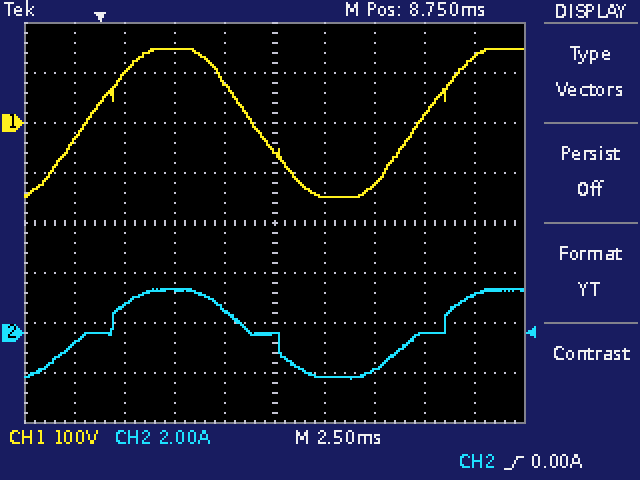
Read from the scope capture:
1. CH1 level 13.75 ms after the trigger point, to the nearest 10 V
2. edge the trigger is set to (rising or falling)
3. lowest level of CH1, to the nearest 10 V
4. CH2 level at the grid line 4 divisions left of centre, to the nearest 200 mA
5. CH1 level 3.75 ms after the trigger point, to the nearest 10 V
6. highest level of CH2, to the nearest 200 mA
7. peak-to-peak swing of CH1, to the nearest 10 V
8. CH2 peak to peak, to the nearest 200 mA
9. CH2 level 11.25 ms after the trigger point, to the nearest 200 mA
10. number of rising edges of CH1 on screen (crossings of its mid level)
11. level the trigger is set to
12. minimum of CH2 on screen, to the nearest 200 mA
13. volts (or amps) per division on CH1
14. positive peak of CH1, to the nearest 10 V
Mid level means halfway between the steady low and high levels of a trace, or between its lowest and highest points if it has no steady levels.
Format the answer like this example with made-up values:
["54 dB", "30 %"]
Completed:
["-120 V", "rising", "-150 V", "-400 mA", "150 V", "1.8 A", "300 V", "3.6 A", "-1.8 A", "2", "0.00 A", "-1.8 A", "100 V", "150 V"]
